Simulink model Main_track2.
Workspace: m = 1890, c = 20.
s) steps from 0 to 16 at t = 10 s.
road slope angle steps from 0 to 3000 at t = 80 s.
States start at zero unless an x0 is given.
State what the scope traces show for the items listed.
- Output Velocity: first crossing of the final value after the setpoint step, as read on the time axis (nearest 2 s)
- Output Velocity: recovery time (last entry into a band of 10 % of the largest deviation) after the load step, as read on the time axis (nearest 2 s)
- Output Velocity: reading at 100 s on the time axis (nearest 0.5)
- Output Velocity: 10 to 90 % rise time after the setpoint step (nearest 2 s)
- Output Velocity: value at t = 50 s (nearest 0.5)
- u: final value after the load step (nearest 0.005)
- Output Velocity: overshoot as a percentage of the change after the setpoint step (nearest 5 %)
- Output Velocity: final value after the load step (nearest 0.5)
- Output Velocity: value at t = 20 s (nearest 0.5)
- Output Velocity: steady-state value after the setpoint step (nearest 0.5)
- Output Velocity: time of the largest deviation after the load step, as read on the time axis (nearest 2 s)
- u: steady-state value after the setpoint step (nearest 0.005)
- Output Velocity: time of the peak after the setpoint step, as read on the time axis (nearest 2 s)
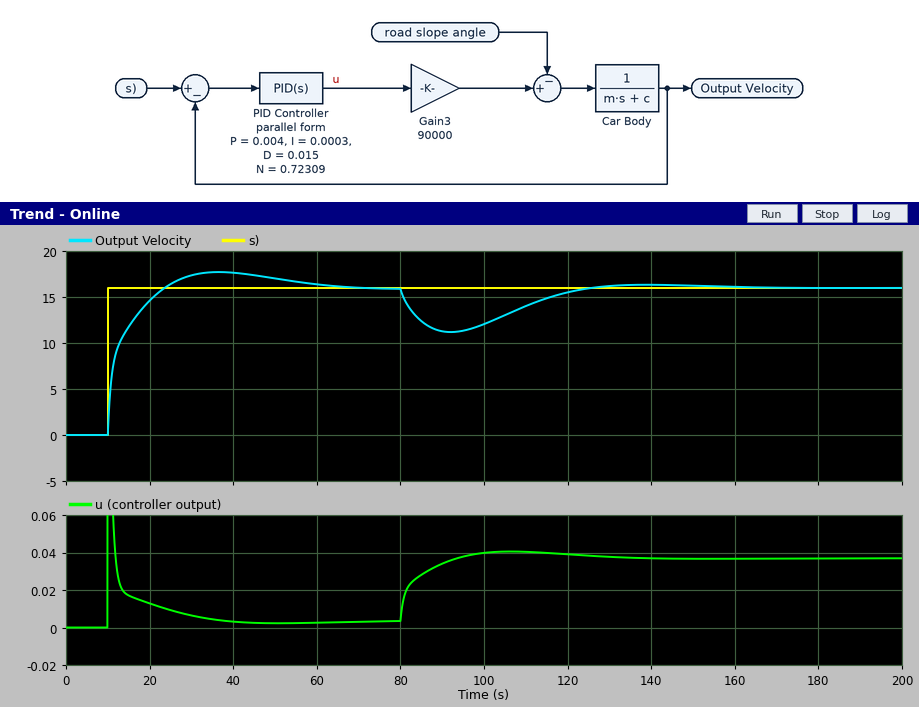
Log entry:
24 s
120 s
12.0
10 s
17.0
0.035
10 %
16.0
14.5
16.0
92 s
0.005
36 s
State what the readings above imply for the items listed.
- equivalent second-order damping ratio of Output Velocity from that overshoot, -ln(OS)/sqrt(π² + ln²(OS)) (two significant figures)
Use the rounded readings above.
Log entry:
0.59
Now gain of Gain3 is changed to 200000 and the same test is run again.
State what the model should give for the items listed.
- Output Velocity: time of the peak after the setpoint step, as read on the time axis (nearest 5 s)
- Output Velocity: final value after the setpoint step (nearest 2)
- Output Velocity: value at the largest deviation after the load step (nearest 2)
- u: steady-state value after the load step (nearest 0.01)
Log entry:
30 s
16
14
0.02
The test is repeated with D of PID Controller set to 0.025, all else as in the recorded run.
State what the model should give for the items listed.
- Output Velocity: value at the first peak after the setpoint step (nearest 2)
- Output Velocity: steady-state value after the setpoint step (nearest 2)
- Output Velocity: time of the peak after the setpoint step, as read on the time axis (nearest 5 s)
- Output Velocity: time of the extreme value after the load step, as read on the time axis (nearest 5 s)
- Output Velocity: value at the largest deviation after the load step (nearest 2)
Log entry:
18
16
40 s
95 s
12
